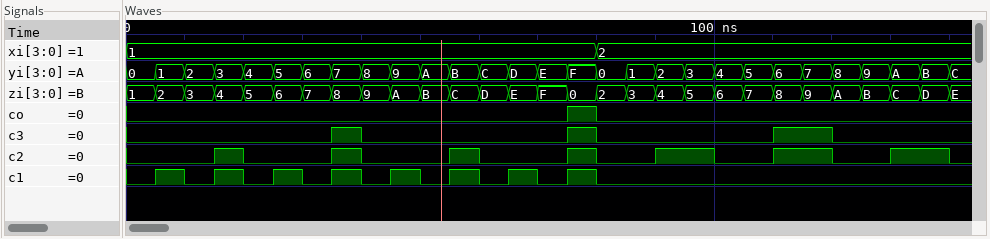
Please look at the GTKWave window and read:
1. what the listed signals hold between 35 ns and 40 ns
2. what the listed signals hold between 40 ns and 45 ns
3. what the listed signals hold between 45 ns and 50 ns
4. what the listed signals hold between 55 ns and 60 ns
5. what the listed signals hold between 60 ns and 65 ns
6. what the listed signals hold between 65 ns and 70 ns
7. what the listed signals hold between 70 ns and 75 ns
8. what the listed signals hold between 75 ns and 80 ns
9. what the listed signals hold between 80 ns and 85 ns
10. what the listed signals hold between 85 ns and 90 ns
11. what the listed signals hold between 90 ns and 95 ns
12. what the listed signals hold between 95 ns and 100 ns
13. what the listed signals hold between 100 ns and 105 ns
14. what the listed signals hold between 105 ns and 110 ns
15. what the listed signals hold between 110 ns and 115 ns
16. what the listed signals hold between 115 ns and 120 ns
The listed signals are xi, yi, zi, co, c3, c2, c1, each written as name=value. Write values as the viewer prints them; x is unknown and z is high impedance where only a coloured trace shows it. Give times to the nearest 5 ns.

xi=1, yi=7, zi=8, co=0, c3=1, c2=1, c1=1
xi=1, yi=8, zi=9, co=0, c3=0, c2=0, c1=0
xi=1, yi=9, zi=A, co=0, c3=0, c2=0, c1=1
xi=1, yi=B, zi=C, co=0, c3=0, c2=1, c1=1
xi=1, yi=C, zi=D, co=0, c3=0, c2=0, c1=0
xi=1, yi=D, zi=E, co=0, c3=0, c2=0, c1=1
xi=1, yi=E, zi=F, co=0, c3=0, c2=0, c1=0
xi=1, yi=F, zi=0, co=1, c3=1, c2=1, c1=1
xi=2, yi=0, zi=2, co=0, c3=0, c2=0, c1=0
xi=2, yi=1, zi=3, co=0, c3=0, c2=0, c1=0
xi=2, yi=2, zi=4, co=0, c3=0, c2=1, c1=0
xi=2, yi=3, zi=5, co=0, c3=0, c2=1, c1=0
xi=2, yi=4, zi=6, co=0, c3=0, c2=0, c1=0
xi=2, yi=5, zi=7, co=0, c3=0, c2=0, c1=0
xi=2, yi=6, zi=8, co=0, c3=1, c2=1, c1=0
xi=2, yi=7, zi=9, co=0, c3=1, c2=1, c1=0
